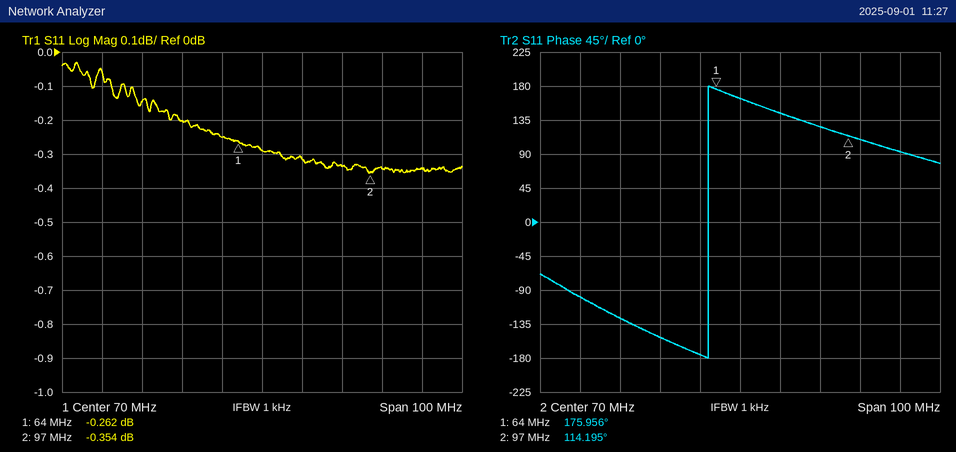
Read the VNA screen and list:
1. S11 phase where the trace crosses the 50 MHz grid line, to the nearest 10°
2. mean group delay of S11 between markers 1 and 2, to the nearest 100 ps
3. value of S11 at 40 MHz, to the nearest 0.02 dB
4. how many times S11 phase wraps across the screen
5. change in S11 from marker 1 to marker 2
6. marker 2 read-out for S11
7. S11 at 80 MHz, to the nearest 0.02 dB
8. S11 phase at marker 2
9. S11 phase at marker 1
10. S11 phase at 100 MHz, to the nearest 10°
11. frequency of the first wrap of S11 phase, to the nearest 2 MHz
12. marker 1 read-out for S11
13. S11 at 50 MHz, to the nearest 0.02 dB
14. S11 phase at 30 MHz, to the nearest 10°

-150°
5.2 ns
-0.14 dB
1
-0.092 dB
-0.354 dB
-0.32 dB
114.195°
175.956°
110°
62 MHz
-0.262 dB
-0.20 dB
-100°
